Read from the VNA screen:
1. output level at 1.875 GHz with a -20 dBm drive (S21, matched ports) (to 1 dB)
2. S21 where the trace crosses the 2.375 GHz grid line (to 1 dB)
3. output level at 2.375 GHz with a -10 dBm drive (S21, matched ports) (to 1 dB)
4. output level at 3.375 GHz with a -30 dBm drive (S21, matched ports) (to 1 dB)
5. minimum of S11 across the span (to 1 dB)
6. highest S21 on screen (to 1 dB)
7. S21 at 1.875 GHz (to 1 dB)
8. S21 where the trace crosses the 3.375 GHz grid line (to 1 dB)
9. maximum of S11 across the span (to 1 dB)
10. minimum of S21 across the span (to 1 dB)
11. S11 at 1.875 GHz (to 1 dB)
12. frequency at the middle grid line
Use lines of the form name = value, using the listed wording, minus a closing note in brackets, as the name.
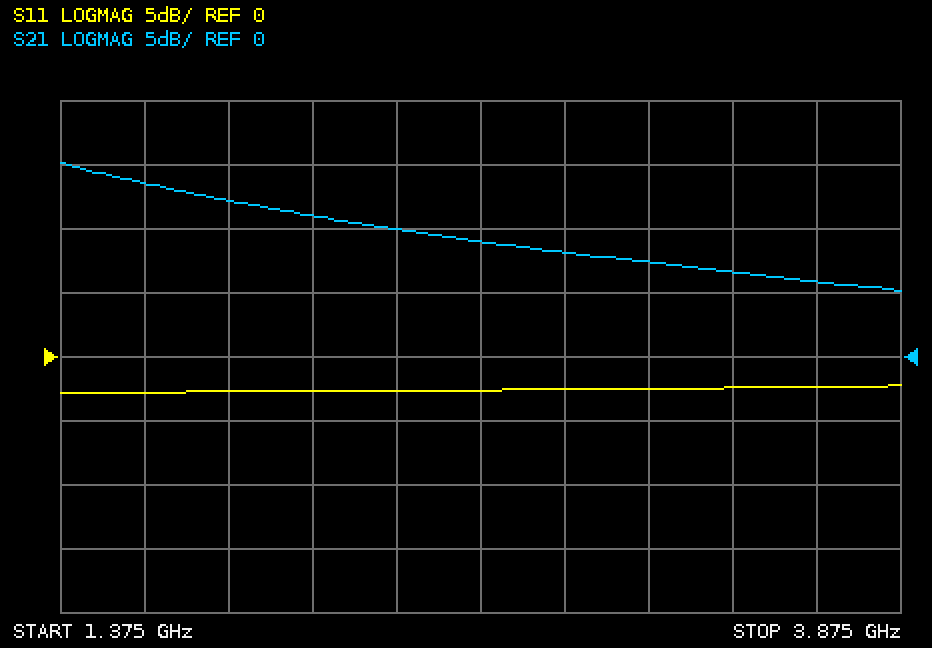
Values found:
output level at 1.875 GHz with a -20 dBm drive (S21, matched ports) = -8 dBm
S21 where the trace crosses the 2.375 GHz grid line = 10 dB
output level at 2.375 GHz with a -10 dBm drive (S21, matched ports) = 0 dBm
output level at 3.375 GHz with a -30 dBm drive (S21, matched ports) = -23 dBm
minimum of S11 across the span = -3 dB
highest S21 on screen = 15 dB
S21 at 1.875 GHz = 12 dB
S21 where the trace crosses the 3.375 GHz grid line = 7 dB
maximum of S11 across the span = -2 dB
minimum of S21 across the span = 5 dB
S11 at 1.875 GHz = -3 dB
frequency at the middle grid line = 2.625 GHz
